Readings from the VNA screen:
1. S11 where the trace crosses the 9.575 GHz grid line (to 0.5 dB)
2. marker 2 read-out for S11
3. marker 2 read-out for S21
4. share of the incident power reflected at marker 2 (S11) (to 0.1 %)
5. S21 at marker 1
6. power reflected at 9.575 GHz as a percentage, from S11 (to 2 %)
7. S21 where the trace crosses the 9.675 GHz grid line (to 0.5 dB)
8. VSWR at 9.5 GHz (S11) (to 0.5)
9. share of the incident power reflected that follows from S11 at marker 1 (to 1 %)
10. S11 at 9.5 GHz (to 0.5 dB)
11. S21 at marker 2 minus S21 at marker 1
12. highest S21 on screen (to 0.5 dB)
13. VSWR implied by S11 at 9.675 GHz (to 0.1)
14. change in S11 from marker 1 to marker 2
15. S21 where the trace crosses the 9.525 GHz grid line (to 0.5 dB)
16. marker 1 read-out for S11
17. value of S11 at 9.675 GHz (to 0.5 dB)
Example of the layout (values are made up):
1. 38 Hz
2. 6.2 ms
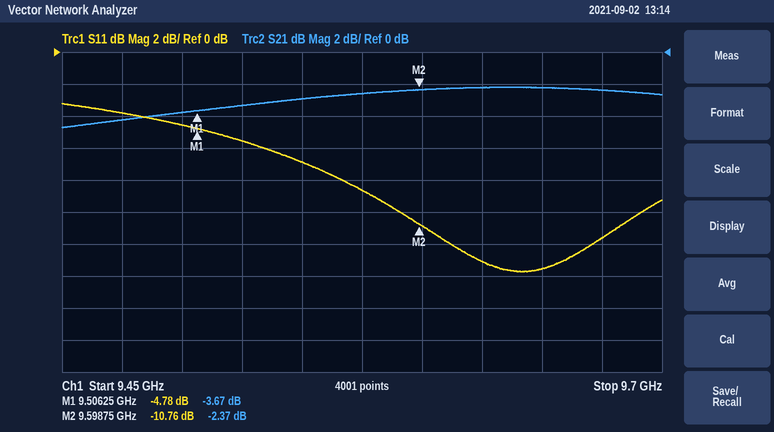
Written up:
1. -8.5 dB
2. -10.76 dB
3. -2.37 dB
4. 8.4 %
5. -3.67 dB
6. 14 %
7. -2.5 dB
8. 4.0
9. 33 %
10. -4.5 dB
11. 1.30 dB
12. -2.0 dB
13. 1.7
14. -5.98 dB
15. -3.5 dB
16. -4.78 dB
17. -11.5 dB
